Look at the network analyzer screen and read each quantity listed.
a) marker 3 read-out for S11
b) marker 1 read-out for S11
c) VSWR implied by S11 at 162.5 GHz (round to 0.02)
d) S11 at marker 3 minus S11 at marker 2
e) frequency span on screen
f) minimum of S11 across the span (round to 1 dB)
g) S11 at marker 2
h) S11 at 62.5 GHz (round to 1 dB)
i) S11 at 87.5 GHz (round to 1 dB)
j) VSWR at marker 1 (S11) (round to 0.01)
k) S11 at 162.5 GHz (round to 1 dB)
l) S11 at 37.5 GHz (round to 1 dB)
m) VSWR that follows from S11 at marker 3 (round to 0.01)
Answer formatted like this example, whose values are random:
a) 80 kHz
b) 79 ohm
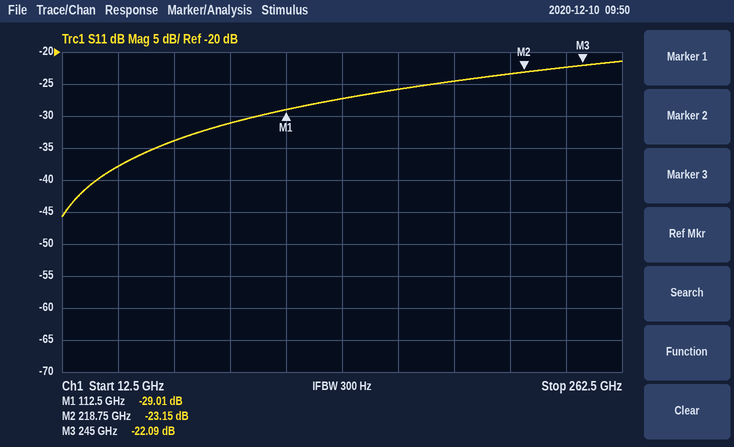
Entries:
a) -22.09 dB
b) -29.01 dB
c) 1.10
d) 1.06 dB
e) 250 GHz
f) -46 dB
g) -23.15 dB
h) -34 dB
i) -31 dB
j) 1.07
k) -26 dB
l) -38 dB
m) 1.17
